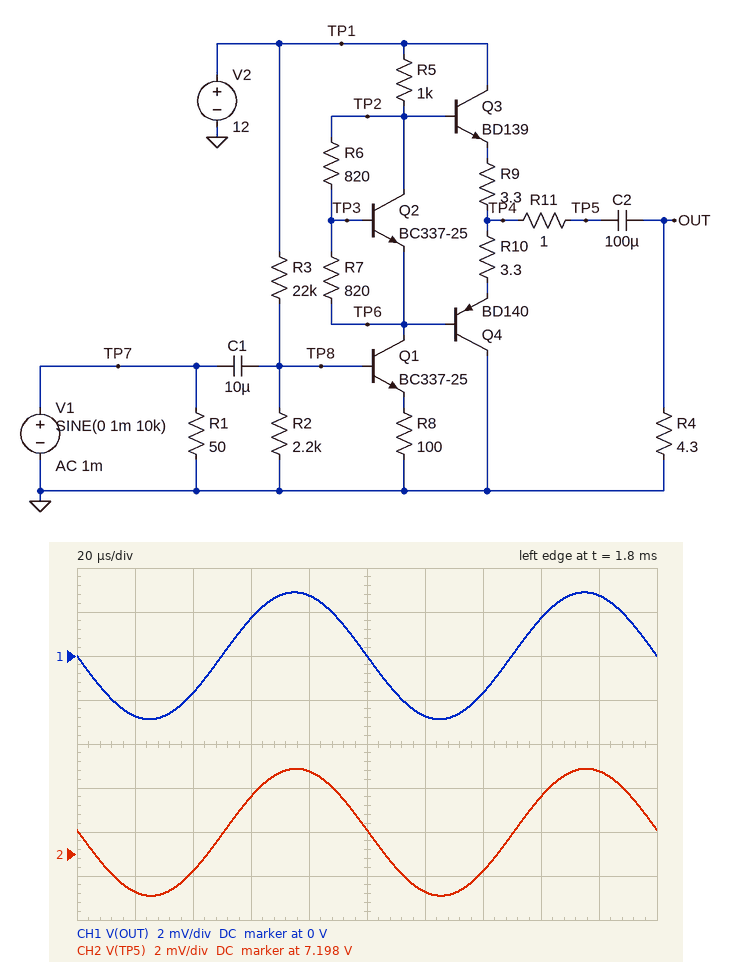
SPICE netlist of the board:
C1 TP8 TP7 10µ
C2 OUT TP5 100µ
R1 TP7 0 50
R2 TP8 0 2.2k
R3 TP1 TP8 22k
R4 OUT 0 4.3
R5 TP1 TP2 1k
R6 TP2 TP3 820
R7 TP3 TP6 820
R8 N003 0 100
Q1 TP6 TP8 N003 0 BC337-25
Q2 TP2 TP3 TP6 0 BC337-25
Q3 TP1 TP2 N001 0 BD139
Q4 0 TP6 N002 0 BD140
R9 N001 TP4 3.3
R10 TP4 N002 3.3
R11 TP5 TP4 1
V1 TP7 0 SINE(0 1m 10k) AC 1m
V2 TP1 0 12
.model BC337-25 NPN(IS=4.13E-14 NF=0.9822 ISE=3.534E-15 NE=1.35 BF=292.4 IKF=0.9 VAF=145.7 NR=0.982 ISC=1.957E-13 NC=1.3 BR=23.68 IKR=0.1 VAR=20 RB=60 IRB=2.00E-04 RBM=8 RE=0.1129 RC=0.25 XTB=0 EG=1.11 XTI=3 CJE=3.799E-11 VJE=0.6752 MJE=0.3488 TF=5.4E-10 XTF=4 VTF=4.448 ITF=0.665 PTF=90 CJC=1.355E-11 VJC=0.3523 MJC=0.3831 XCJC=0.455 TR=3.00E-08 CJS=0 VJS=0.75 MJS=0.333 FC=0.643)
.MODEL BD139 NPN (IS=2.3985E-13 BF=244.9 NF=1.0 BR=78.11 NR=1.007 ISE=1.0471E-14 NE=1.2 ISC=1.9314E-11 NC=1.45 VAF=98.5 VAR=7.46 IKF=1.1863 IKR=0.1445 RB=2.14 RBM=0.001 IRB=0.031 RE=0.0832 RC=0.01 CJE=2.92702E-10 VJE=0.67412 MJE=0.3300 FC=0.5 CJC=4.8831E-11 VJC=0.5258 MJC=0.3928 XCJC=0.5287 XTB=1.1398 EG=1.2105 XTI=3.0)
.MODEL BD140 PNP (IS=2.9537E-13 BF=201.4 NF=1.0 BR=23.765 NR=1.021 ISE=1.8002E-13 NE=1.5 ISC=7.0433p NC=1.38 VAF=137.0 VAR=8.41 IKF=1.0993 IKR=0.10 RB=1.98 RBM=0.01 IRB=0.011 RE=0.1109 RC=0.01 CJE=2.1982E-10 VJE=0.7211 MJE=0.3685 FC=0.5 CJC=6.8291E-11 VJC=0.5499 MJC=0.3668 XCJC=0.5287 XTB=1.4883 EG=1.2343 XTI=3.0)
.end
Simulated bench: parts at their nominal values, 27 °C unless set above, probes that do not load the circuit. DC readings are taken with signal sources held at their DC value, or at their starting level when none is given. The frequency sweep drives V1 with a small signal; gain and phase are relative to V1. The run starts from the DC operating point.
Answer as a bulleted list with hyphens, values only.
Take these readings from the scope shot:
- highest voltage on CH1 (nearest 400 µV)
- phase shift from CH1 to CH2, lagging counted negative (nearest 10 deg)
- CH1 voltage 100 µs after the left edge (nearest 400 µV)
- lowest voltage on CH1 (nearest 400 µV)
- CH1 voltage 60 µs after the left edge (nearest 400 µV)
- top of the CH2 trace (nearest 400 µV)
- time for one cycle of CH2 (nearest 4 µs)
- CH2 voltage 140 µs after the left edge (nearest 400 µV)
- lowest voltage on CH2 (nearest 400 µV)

- 2.8 mV
- 0 deg
- 0 V
- -2.8 mV
- 1.6 mV
- 7.2020 V
- 100 µs
- 7.1972 V
- 7.1960 V
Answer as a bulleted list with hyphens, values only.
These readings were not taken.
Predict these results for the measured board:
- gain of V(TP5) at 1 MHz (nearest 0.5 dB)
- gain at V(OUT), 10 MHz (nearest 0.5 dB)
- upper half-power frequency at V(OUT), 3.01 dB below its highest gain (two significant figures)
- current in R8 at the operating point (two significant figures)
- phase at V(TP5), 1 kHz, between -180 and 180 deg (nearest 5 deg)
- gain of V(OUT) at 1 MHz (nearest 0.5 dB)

- 6.5 dB
- -10.0 dB
- 1.1 MHz
- 4.2 mA
- 165 deg
- 6.5 dB
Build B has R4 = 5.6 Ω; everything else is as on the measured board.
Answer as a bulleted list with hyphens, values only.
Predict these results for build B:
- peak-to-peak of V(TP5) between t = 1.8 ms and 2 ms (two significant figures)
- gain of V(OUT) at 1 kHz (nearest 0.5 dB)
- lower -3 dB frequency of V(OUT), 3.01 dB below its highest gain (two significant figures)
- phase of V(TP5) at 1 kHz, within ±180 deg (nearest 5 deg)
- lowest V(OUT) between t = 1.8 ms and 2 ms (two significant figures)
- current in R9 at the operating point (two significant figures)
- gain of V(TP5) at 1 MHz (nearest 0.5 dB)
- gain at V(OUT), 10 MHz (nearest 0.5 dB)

- 6.9 mV
- 10.5 dB
- 100 Hz
- 170 deg
- -3.4 mV
- 6.9 mA
- 8.5 dB
- -8.0 dB
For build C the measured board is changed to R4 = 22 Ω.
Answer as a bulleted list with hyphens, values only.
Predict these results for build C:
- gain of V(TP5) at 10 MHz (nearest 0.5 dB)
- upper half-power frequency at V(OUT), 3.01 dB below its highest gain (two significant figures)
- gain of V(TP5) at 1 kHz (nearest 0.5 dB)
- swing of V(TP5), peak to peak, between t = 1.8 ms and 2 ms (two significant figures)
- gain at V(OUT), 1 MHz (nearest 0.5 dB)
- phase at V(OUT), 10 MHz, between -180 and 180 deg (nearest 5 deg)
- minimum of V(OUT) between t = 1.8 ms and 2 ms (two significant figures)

- 1.0 dB
- 1.7 MHz
- 16.5 dB
- 13 mV
- 15.0 dB
- 100 deg
- -6.5 mV
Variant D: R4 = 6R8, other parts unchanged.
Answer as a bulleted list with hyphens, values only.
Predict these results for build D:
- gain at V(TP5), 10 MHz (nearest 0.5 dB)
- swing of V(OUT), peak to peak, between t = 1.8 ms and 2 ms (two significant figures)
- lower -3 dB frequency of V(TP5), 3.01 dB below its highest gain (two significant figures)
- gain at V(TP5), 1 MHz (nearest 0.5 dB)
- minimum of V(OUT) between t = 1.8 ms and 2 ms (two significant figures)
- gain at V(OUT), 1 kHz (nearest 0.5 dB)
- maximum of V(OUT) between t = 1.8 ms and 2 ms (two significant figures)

- -6.5 dB
- 7.7 mV
- 7.4 Hz
- 9.5 dB
- -3.9 mV
- 11.5 dB
- 3.9 mV
